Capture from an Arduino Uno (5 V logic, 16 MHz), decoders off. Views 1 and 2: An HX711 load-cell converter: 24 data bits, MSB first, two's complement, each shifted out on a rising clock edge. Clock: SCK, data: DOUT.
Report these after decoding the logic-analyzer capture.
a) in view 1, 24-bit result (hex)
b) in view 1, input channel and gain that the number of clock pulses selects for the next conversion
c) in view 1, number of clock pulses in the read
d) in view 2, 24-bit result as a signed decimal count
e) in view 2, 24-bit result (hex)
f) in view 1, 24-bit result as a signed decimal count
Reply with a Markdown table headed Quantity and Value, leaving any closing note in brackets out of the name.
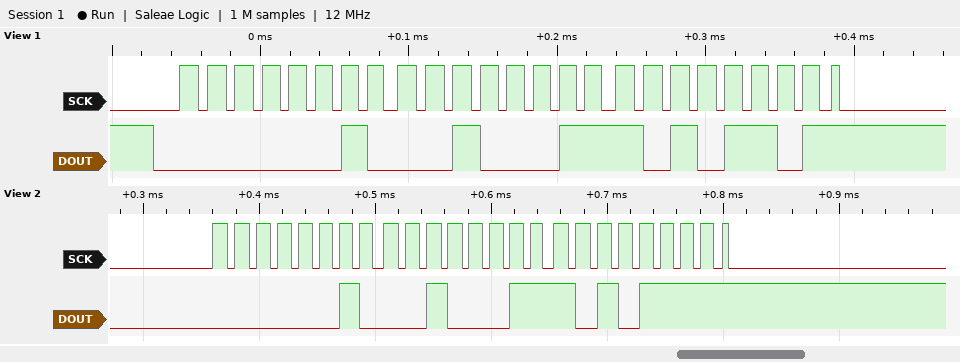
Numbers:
| Quantity | Value |
|---|---|
| in view 1, 24-bit result | 0x0223AD |
| in view 1, input channel and gain that the number of clock pulses selects for the next conversion | channel A, gain 128 |
| in view 1, number of clock pulses in the read | 25 |
| in view 2, 24-bit result as a signed decimal count | 140207 |
| in view 2, 24-bit result | 0x0223AF |
| in view 1, 24-bit result as a signed decimal count | 140205 |
